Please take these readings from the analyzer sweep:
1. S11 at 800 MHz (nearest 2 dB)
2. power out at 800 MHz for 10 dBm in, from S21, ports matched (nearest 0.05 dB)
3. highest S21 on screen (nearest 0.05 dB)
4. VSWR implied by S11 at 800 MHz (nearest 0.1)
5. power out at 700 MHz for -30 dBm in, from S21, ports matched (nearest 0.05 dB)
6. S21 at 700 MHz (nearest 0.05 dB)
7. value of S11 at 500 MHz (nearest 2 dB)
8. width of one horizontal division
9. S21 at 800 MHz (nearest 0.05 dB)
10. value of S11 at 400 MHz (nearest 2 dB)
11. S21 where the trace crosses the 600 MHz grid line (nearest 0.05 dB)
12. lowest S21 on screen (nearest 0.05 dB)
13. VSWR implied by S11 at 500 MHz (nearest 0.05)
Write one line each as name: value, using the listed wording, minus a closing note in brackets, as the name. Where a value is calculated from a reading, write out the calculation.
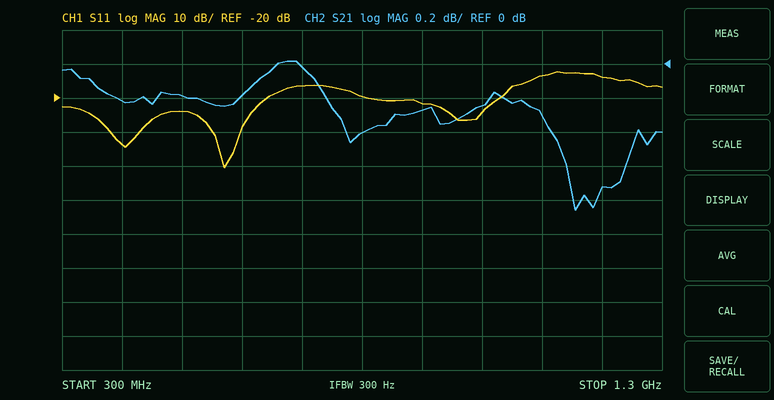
S11 at 800 MHz: -20 dB
power out at 800 MHz for 10 dBm in, from S21, ports matched: 10 dBm + (-0.40 dB) = 9.60 dBm
highest S21 on screen: 0.00 dB
VSWR implied by S11 at 800 MHz: |Γ| = 10^(-20/20) = 0.1000; VSWR = (1 + 0.1000)/(1 − 0.1000) ≈ 1.2
power out at 700 MHz for -30 dBm in, from S21, ports matched: -30 dBm + (0.00 dB) = -30.00 dBm
S21 at 700 MHz: 0.00 dB
value of S11 at 500 MHz: -24 dB
width of one horizontal division: 100 MHz
S21 at 800 MHz: -0.40 dB
value of S11 at 400 MHz: -34 dB
S21 where the trace crosses the 600 MHz grid line: -0.20 dB
lowest S21 on screen: -0.85 dB
VSWR implied by S11 at 500 MHz: |Γ| = 10^(-24/20) = 0.0631; VSWR = (1 + 0.0631)/(1 − 0.0631) ≈ 1.13, so 1.15 to the nearest 0.05
